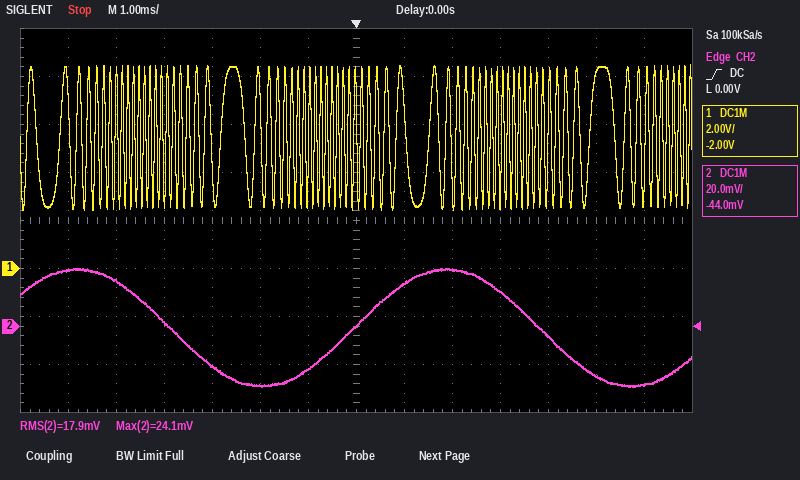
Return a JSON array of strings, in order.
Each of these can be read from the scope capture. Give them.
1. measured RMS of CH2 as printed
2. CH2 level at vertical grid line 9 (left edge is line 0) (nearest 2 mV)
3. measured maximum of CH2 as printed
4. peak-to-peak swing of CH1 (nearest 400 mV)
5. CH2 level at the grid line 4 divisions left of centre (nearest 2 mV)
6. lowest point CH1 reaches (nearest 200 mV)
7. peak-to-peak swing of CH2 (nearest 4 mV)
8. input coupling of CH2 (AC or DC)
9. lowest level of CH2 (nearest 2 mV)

["17.9 mV", "24 mV", "24.1 mV", "6.0 V", "2 mV", "2.4 V", "48 mV", "DC", "-26 mV"]
